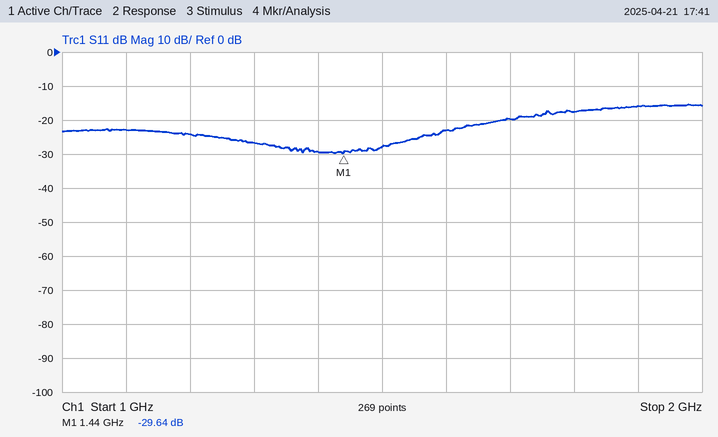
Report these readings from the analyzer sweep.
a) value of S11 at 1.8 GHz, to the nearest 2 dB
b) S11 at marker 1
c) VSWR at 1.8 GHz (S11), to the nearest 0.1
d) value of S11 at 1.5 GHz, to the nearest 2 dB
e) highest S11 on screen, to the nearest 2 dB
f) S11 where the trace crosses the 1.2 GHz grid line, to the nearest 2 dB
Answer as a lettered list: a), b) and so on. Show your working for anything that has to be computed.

a) -18 dB
b) -29.64 dB
c) |Γ| = 10^(-18/20) = 0.1259; VSWR = (1 + 0.1259)/(1 − 0.1259) ≈ 1.3
d) -28 dB
e) -16 dB
f) -24 dB
